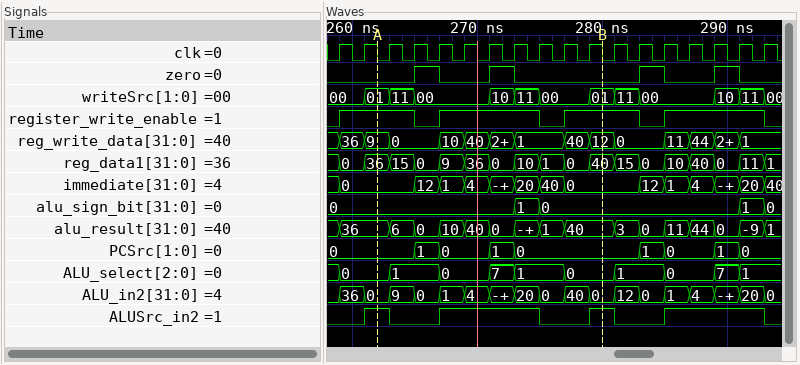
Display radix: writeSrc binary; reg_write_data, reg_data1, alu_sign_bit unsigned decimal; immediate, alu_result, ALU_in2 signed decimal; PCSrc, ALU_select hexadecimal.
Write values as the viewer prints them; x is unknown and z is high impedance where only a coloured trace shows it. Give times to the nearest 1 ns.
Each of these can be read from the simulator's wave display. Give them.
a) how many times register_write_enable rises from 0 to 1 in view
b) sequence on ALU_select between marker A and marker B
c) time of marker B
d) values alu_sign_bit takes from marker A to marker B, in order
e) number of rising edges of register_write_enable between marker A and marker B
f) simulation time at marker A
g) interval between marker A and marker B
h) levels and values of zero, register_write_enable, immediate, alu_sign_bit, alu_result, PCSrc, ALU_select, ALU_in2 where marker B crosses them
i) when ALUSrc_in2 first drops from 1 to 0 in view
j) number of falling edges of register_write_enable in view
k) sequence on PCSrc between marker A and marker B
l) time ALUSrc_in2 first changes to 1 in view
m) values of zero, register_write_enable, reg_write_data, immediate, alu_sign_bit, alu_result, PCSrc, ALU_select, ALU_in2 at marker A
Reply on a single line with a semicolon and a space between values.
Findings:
4; 0, 1, 0, 7, 1, 0; 280 ns; 0, 1, 0; 2; 262 ns; 18 ns; zero=0, register_write_enable=1, immediate=0, alu_sign_bit=0, alu_result=40, PCSrc=0, ALU_select=0, ALU_in2=0; 263 ns; 4; 0, 1, 0, 1, 0; 261 ns; zero=0, register_write_enable=1, reg_write_data=9, immediate=0, alu_sign_bit=0, alu_result=36, PCSrc=0, ALU_select=0, ALU_in2=0
